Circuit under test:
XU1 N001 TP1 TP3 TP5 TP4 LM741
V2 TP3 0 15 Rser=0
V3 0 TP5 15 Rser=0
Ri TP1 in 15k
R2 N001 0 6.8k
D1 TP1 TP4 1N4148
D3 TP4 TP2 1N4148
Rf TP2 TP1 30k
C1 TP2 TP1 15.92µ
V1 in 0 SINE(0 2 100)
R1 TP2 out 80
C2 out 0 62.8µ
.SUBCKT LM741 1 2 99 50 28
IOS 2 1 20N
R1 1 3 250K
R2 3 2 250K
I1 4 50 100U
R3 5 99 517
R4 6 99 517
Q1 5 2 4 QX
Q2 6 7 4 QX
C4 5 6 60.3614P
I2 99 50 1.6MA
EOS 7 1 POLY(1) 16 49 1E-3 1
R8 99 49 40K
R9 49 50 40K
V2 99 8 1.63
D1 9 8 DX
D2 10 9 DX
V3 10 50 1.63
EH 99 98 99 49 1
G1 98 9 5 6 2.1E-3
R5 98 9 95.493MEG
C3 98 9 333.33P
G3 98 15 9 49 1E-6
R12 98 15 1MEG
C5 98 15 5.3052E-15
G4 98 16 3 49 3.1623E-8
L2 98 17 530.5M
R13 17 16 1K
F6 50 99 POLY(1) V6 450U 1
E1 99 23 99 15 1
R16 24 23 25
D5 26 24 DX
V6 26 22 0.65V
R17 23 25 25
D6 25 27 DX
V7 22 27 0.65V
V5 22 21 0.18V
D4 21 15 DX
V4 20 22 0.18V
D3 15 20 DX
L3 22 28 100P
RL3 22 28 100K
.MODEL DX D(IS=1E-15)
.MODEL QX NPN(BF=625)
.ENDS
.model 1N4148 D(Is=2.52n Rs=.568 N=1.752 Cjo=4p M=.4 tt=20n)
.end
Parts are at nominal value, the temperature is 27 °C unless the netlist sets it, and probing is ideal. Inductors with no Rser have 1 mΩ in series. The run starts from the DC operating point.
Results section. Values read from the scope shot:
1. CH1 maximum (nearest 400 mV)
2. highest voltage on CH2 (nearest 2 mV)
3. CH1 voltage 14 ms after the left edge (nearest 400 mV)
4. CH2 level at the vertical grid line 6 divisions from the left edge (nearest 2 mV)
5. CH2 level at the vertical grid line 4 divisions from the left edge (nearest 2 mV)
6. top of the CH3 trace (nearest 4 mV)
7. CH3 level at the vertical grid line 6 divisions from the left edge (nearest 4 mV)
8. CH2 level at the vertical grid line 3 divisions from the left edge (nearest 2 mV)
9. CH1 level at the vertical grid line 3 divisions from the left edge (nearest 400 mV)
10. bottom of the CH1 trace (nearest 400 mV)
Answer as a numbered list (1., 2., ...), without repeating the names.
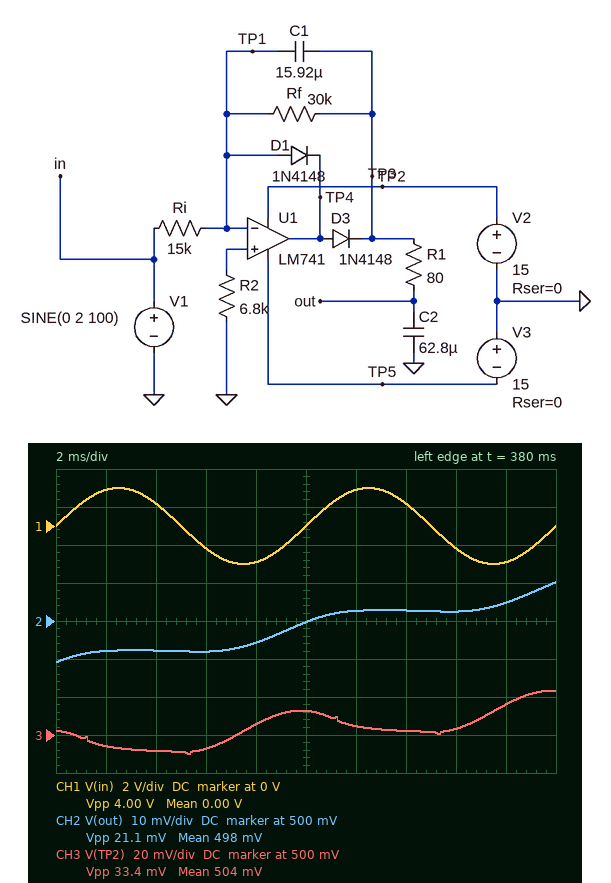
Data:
1. 2.0 V
2. 510 mV
3. 1.2 V
4. 502 mV
5. 494 mV
6. 524 mV
7. 504 mV
8. 492 mV
9. -1.2 V
10. -2.0 V
